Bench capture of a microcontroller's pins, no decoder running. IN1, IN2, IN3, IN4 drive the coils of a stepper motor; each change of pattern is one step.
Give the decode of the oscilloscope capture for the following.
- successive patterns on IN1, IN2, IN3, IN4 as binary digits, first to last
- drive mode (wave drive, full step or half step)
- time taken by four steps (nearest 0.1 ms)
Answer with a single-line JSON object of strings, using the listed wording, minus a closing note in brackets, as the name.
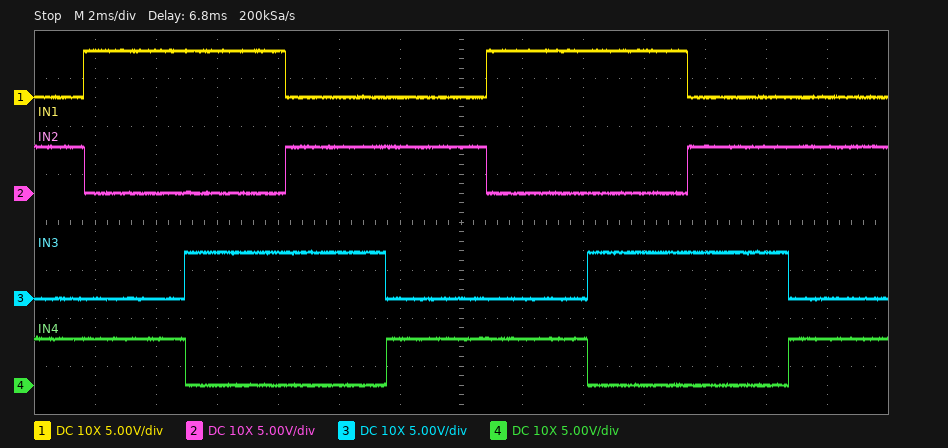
{"successive patterns on IN1, IN2, IN3, IN4 as binary digits, first to last": "0101 1001 1010 0110 0101 1001 1010 0110 0101", "drive mode": "full step", "time taken by four steps": "13.2 ms"}
